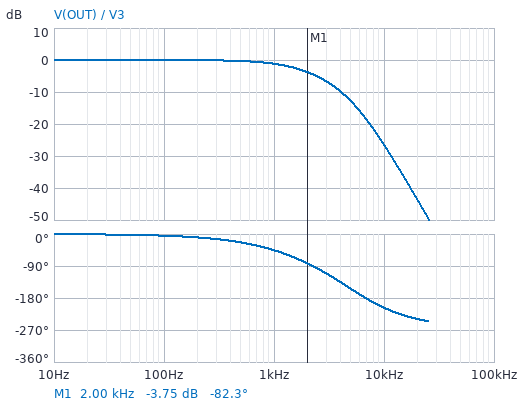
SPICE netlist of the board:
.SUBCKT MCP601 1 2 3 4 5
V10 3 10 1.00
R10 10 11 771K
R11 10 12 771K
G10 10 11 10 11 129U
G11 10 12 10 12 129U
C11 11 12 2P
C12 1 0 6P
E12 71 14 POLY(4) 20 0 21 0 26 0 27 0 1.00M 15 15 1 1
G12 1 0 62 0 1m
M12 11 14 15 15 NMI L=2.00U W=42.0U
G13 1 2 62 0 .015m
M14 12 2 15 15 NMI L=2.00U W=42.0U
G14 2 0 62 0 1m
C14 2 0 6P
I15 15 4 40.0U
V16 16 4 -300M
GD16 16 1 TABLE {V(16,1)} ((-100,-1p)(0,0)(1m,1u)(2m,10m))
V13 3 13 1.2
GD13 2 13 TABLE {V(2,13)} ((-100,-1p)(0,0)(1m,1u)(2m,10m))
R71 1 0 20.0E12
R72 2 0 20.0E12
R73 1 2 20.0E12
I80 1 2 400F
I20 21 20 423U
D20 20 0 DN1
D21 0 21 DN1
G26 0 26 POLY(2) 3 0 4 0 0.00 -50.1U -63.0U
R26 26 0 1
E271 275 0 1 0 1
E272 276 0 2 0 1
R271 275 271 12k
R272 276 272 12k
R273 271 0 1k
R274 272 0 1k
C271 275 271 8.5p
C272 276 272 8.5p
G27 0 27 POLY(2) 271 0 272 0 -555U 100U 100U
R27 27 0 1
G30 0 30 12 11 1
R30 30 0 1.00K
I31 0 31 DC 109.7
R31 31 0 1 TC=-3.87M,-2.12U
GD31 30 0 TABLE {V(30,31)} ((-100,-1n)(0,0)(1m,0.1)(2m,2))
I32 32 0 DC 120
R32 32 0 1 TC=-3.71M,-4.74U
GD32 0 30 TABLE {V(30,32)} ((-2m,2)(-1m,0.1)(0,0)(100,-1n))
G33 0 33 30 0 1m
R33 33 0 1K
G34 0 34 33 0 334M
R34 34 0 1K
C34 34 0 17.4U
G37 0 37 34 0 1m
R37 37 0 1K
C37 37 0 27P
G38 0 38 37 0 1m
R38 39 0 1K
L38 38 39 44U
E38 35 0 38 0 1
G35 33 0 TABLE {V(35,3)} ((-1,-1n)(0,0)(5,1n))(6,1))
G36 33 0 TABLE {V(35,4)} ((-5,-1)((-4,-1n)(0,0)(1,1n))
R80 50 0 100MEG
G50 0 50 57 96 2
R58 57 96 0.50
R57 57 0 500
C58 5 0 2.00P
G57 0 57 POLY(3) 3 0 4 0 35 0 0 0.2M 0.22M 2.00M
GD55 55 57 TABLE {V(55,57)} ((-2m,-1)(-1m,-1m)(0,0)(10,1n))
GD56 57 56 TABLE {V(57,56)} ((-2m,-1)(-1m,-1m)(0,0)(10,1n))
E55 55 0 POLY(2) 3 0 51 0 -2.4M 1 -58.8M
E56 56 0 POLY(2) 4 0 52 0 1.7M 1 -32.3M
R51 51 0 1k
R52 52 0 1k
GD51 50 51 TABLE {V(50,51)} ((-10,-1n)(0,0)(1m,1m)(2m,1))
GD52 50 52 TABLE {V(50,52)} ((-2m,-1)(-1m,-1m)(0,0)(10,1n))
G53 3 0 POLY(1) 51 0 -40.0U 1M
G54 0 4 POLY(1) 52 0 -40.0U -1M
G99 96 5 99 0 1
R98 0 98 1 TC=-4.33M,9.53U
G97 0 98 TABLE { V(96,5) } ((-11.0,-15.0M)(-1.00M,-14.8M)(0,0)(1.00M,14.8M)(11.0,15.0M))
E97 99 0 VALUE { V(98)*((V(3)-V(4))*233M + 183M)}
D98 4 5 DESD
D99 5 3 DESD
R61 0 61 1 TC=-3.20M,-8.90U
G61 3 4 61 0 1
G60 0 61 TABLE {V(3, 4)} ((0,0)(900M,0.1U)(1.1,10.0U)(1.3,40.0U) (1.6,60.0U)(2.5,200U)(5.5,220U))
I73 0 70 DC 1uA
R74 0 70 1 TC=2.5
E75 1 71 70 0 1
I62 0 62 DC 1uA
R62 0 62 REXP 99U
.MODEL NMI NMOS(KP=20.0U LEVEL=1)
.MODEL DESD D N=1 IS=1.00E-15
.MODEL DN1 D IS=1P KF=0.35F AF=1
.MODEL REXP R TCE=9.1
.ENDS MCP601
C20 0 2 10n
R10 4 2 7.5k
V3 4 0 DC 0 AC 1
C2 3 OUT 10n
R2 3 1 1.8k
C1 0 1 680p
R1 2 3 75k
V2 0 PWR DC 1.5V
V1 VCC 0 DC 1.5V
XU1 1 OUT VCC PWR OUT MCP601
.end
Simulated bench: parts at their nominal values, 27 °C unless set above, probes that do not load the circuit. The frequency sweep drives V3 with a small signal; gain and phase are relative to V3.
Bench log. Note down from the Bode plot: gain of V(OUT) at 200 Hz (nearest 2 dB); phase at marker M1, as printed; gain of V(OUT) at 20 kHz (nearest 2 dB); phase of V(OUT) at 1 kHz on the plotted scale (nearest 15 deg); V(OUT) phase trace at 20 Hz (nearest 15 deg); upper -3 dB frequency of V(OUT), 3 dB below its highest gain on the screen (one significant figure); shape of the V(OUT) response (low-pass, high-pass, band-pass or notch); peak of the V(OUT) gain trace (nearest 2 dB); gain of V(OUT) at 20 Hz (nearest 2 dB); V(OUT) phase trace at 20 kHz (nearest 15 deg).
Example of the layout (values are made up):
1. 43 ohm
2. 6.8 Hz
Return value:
1. 0 dB
2. -82.3 deg
3. -44 dB
4. -45 deg
5. 0 deg
6. 2 kHz
7. low-pass
8. 0 dB
9. 0 dB
10. -240 deg
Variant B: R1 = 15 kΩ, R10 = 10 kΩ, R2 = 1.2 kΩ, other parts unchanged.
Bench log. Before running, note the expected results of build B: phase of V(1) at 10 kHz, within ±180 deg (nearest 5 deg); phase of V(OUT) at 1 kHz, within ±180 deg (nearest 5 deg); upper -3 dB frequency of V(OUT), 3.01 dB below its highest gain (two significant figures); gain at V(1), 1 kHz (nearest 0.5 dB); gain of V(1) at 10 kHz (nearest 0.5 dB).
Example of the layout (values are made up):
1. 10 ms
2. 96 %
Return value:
1. -135 deg
2. -40 deg
3. 1.5 kHz
4. -1.5 dB
5. -15.5 dB
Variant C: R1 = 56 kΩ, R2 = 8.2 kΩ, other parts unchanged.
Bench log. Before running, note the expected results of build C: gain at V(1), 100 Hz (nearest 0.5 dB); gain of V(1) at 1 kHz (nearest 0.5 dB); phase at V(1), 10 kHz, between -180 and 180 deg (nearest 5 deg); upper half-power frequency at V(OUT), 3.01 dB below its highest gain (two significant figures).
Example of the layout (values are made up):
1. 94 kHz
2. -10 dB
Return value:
1. 0 dB
2. 0 dB
3. 115 deg
4. 2.8 kHz
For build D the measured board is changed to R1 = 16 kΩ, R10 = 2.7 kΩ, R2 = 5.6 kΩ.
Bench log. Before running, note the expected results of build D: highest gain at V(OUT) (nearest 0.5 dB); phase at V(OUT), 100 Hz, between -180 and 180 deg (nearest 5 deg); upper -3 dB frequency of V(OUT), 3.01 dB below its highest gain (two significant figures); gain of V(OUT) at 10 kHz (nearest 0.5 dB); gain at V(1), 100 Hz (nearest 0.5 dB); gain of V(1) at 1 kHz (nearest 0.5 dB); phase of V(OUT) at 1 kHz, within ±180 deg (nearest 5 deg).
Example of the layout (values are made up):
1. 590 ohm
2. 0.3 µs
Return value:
1. 1.5 dB
2. 0 deg
3. 6.8 kHz
4. -11.5 dB
5. 0 dB
6. 0 dB
7. -15 deg
